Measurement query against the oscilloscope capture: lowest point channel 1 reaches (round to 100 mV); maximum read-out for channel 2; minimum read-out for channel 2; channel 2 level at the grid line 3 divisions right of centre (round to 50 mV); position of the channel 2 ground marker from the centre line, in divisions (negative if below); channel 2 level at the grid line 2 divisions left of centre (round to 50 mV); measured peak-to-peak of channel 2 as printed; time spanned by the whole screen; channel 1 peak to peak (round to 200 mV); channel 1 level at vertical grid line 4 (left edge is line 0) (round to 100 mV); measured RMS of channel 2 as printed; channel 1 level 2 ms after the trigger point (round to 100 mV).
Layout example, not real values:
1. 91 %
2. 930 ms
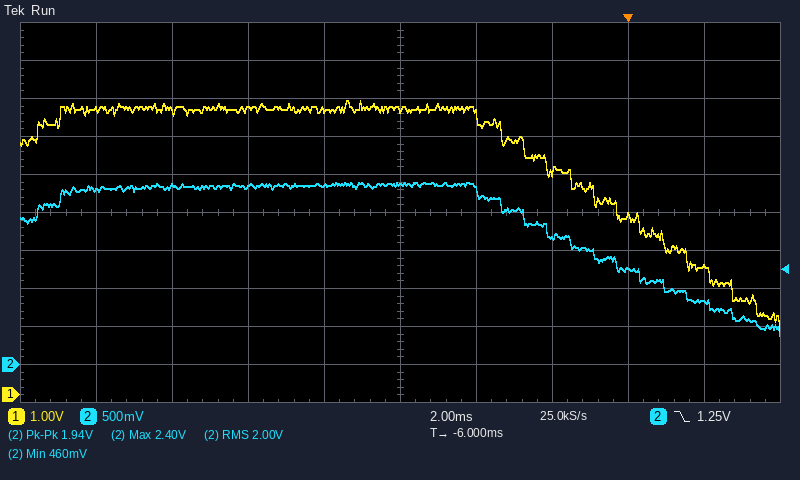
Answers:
1. 1.7 V
2. 2.40 V
3. 460 mV
4. 1.25 V
5. -4.0 div
6. 2.35 V
7. 1.94 V
8. 20 ms
9. 6.0 V
10. 7.5 V
11. 2.00 V
12. 3.4 V
